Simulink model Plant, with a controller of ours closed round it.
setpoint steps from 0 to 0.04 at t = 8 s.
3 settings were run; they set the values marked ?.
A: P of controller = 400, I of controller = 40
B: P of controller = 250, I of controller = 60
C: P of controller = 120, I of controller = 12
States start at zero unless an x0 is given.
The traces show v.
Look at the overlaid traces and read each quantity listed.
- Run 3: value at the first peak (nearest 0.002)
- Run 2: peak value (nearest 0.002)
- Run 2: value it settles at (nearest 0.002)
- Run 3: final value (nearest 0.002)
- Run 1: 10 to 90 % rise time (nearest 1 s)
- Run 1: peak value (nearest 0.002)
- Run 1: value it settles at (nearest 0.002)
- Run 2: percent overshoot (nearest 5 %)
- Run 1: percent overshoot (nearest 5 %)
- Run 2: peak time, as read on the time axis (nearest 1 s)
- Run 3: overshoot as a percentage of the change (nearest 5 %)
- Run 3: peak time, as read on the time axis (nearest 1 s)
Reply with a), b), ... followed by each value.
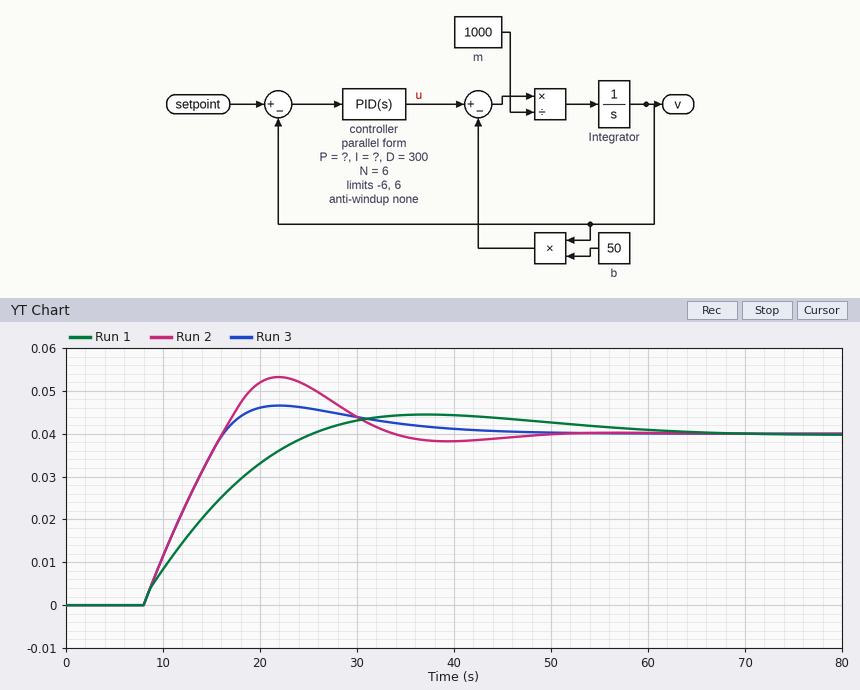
a) 0.046
b) 0.054
c) 0.040
d) 0.040
e) 13 s
f) 0.044
g) 0.040
h) 35 %
i) 10 %
j) 22 s
k) 15 %
l) 22 s
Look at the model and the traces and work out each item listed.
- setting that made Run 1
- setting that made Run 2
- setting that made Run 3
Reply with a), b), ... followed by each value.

a) C
b) B
c) A
